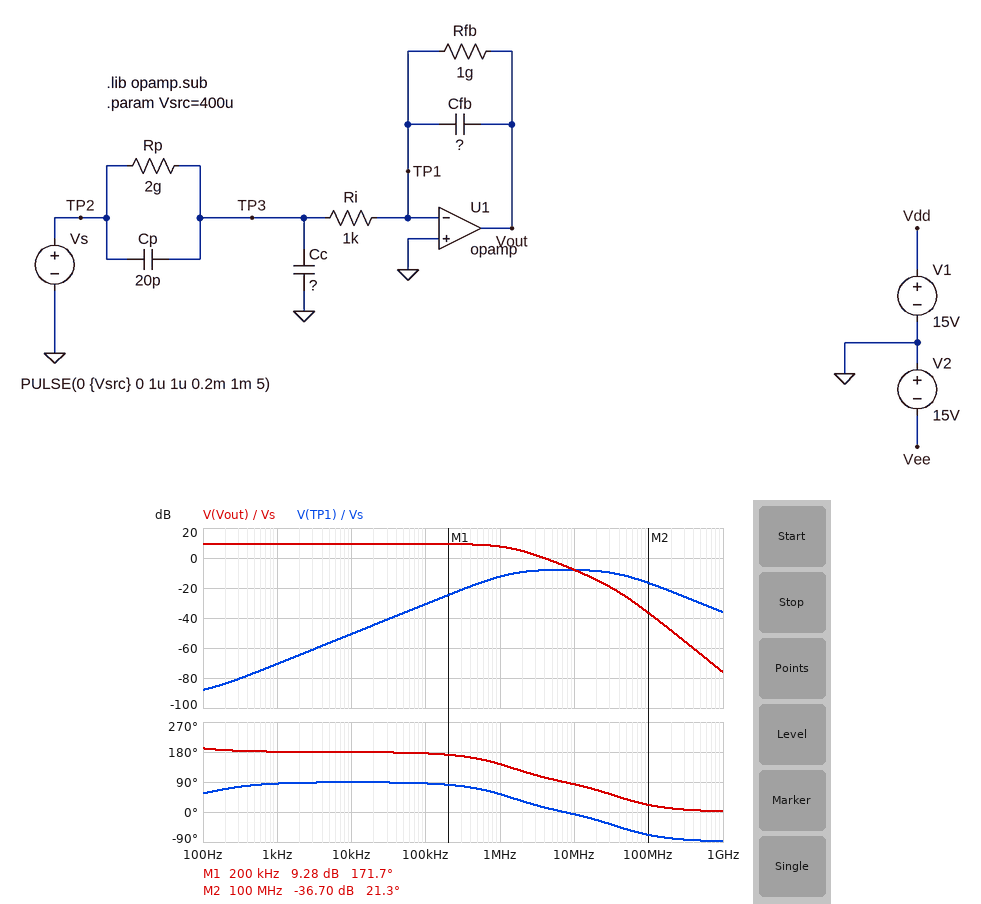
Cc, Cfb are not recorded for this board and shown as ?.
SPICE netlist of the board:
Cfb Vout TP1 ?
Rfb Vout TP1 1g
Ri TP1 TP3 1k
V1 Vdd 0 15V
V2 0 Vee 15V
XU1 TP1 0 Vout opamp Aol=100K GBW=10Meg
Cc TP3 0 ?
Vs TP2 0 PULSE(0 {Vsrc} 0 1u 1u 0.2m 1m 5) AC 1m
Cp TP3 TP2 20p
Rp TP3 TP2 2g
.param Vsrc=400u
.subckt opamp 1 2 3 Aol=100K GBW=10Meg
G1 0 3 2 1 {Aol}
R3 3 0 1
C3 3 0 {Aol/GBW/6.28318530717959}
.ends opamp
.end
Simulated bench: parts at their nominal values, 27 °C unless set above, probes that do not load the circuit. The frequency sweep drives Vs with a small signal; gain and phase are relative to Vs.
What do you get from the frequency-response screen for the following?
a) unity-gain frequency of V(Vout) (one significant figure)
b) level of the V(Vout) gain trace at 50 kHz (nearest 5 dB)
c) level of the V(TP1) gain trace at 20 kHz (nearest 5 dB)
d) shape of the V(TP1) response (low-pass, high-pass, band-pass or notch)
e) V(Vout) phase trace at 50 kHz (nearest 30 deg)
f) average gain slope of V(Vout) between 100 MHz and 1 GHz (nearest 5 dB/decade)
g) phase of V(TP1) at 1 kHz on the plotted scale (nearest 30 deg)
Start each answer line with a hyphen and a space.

- 4 MHz
- 10 dB
- -45 dB
- band-pass
- 180 deg
- -40 dB/decade
- 90 deg
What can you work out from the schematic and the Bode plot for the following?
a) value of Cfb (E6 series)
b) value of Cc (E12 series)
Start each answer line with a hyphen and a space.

- 6.8 pF
- 10 pF
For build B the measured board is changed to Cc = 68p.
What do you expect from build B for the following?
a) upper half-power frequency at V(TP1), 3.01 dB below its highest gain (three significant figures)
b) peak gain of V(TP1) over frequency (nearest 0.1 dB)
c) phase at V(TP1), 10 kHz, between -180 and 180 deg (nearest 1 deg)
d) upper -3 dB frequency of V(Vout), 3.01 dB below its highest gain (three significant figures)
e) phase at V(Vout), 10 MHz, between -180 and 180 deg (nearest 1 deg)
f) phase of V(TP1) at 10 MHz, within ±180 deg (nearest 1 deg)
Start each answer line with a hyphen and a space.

- 35.7 MHz
- -16.4 dB
- 88 deg
- 521 kHz
- 77 deg
- -13 deg
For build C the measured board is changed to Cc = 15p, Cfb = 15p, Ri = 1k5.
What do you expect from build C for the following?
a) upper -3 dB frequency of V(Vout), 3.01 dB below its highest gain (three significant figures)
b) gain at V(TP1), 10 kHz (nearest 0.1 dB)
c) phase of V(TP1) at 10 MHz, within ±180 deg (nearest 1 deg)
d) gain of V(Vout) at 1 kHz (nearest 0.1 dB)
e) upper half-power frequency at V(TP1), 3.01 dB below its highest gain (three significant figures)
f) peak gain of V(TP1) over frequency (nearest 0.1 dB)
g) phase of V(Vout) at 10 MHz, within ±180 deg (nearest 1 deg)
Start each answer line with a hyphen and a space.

- 1.63 MHz
- -57.5 dB
- -19 deg
- 2.5 dB
- 21.5 MHz
- -13.9 dB
- 71 deg
